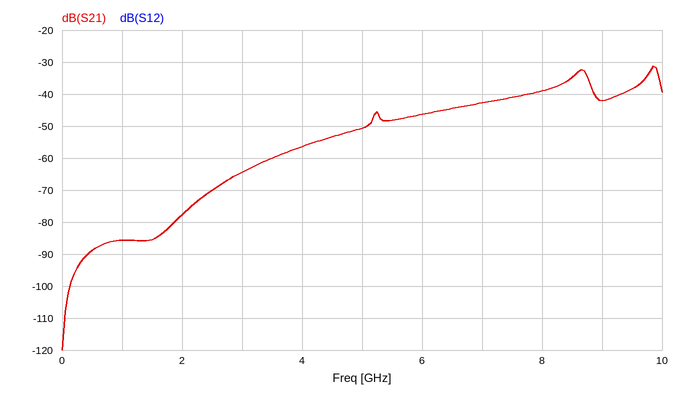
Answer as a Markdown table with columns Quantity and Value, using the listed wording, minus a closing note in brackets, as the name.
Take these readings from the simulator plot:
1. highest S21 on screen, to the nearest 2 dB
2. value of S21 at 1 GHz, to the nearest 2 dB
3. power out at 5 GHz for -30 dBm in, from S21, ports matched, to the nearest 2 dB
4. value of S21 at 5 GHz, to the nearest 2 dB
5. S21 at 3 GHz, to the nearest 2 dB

| Quantity | Value |
|---|---|
| highest S21 on screen, to the nearest 2 dB | -32 dB |
| value of S21 at 1 GHz, to the nearest 2 dB | -86 dB |
| power out at 5 GHz for -30 dBm in, from S21, ports matched, to the nearest 2 dB | -80 dBm |
| value of S21 at 5 GHz, to the nearest 2 dB | -50 dB |
| S21 at 3 GHz, to the nearest 2 dB | -64 dB |
